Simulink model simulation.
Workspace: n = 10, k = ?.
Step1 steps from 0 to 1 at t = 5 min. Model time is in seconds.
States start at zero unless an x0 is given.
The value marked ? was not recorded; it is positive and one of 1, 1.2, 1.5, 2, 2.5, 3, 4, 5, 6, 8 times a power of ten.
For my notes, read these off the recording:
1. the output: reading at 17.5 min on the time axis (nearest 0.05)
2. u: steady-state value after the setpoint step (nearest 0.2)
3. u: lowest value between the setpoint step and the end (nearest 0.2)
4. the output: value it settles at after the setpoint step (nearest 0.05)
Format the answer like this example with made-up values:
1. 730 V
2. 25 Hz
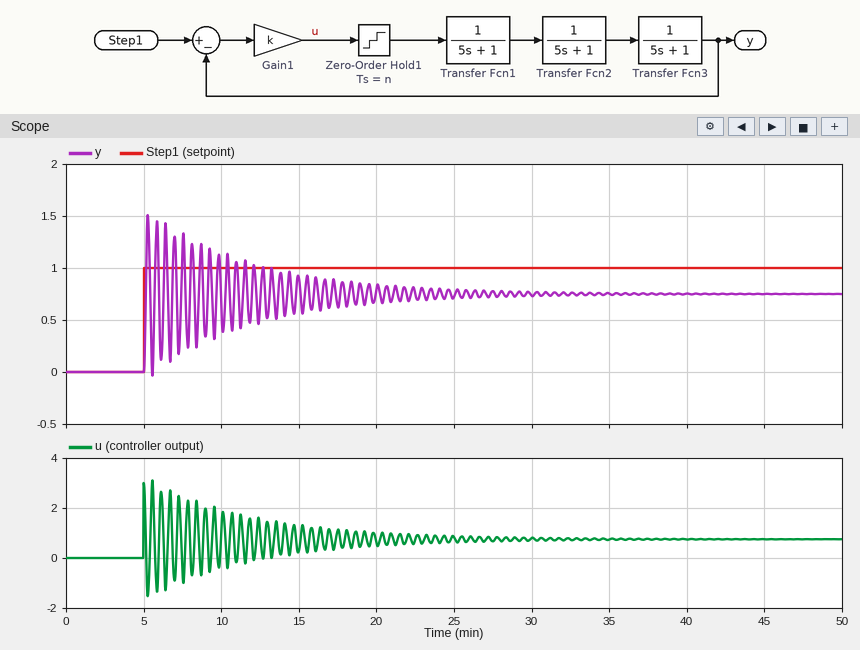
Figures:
1. 0.65
2. 0.8
3. -1.6
4. 0.75
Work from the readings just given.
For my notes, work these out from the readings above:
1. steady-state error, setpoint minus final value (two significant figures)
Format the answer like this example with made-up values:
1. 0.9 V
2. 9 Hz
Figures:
1. 0.25
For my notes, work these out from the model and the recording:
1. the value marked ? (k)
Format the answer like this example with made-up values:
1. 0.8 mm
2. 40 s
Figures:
1. 3
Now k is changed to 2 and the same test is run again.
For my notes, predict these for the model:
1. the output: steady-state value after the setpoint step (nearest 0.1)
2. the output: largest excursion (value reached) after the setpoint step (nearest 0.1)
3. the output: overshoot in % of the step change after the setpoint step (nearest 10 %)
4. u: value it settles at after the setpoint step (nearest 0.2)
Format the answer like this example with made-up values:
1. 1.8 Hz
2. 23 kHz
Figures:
1. 0.7
2. 1.1
3. 70 %
4. 0.6
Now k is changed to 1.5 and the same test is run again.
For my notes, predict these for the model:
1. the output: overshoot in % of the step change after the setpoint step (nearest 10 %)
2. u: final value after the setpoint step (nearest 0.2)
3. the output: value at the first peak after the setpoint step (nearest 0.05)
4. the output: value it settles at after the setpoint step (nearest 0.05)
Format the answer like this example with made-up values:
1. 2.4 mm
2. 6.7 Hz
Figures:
1. 50 %
2. 0.6
3. 0.90
4. 0.60
